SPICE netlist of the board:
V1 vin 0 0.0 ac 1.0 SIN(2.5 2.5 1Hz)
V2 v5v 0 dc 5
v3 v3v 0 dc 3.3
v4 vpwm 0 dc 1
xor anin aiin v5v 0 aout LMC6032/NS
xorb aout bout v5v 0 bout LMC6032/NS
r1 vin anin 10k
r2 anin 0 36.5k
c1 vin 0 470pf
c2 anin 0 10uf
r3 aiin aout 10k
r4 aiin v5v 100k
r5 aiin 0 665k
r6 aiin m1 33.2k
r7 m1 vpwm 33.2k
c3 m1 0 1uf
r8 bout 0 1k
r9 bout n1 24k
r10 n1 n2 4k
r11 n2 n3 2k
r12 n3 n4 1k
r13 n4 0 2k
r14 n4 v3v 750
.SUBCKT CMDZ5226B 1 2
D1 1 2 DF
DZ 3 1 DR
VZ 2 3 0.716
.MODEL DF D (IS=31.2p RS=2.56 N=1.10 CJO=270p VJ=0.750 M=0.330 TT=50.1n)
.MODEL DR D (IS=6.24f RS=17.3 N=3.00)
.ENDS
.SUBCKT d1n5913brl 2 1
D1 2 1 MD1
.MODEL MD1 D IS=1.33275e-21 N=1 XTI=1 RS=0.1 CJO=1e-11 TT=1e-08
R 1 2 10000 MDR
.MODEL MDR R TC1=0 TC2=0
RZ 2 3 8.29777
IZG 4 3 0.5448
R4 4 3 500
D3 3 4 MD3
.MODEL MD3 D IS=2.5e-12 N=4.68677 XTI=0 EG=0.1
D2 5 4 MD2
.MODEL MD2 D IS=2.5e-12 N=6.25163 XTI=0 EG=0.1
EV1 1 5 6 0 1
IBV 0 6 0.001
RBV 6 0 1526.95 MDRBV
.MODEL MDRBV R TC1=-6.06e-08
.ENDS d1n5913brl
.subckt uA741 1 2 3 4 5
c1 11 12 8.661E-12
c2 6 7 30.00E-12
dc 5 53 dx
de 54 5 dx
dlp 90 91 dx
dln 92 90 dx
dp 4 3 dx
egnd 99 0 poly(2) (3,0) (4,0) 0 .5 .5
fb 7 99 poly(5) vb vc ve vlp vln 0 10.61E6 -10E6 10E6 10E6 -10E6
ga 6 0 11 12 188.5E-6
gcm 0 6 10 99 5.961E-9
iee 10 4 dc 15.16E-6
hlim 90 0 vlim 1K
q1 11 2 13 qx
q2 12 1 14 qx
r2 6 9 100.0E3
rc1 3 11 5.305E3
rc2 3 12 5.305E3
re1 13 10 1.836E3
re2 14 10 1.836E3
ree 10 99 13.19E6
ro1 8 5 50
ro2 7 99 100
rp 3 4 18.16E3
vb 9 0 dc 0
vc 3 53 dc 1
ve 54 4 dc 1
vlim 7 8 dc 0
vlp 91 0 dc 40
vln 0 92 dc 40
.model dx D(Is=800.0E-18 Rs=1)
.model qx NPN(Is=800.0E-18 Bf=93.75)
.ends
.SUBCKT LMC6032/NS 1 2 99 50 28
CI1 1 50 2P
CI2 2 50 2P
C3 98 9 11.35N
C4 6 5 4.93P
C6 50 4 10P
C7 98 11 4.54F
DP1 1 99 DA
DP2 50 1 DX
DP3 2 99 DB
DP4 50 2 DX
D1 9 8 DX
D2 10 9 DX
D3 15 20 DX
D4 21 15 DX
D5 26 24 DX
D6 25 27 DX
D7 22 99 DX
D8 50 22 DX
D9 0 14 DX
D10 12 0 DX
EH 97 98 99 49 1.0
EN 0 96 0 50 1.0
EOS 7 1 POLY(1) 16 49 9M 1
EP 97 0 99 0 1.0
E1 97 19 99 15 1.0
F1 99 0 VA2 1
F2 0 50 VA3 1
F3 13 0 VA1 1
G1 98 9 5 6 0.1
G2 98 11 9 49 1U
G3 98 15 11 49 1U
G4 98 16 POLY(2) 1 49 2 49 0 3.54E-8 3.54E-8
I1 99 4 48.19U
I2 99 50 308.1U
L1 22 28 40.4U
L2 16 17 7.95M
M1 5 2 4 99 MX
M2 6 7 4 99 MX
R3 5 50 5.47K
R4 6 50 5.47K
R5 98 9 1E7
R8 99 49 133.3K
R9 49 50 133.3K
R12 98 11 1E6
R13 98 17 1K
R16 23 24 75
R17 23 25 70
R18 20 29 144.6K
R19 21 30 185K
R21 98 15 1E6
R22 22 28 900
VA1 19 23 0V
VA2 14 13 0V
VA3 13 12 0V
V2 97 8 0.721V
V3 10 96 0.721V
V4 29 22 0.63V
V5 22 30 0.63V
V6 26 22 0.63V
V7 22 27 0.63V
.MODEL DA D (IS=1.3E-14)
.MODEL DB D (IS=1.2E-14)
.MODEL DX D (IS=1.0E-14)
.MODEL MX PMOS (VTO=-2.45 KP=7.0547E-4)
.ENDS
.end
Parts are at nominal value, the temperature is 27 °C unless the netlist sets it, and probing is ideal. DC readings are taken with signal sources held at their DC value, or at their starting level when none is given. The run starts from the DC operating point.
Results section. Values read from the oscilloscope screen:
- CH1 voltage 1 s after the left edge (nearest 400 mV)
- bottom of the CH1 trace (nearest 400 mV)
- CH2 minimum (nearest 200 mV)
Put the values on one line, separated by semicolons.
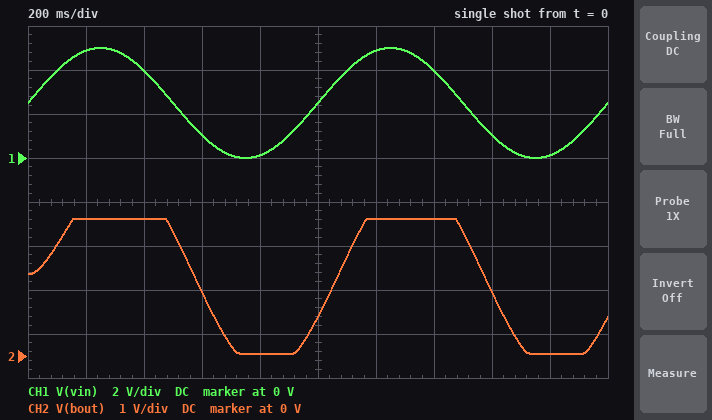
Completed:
2.4 V; 0 V; 0 V
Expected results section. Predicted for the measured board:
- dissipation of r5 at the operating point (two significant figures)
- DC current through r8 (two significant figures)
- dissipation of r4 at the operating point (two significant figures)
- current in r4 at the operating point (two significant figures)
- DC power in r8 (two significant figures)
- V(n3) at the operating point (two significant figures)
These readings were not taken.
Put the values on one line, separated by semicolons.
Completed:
380 nW; 35 µA; 200 µW; 45 µA; 1.2 µW; 2.3 V
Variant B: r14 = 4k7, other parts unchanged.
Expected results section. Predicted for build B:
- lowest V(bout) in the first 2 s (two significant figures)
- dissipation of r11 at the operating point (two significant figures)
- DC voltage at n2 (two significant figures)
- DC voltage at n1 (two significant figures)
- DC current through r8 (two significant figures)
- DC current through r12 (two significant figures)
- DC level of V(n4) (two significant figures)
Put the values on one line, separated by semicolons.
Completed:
33 mV; 1.7 µW; 860 mV; 740 mV; 32 µA; 29 µA; 940 mV
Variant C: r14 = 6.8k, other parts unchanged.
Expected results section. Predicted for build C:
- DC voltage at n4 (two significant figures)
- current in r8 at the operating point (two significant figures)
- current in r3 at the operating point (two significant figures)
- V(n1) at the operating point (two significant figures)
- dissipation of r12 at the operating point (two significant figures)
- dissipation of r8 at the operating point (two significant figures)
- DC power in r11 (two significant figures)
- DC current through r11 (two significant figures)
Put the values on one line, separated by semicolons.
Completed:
720 mV; 32 µA; 52 µA; 560 mV; 490 nW; 1.0 µW; 970 nW; 22 µA
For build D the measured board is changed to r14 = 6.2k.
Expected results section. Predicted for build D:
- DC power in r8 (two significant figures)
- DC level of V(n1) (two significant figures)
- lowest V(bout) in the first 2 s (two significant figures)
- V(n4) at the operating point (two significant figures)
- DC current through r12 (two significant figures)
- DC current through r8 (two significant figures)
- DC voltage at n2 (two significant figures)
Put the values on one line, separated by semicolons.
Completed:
1.0 µW; 600 mV; 33 mV; 770 mV; 24 µA; 32 µA; 700 mV
